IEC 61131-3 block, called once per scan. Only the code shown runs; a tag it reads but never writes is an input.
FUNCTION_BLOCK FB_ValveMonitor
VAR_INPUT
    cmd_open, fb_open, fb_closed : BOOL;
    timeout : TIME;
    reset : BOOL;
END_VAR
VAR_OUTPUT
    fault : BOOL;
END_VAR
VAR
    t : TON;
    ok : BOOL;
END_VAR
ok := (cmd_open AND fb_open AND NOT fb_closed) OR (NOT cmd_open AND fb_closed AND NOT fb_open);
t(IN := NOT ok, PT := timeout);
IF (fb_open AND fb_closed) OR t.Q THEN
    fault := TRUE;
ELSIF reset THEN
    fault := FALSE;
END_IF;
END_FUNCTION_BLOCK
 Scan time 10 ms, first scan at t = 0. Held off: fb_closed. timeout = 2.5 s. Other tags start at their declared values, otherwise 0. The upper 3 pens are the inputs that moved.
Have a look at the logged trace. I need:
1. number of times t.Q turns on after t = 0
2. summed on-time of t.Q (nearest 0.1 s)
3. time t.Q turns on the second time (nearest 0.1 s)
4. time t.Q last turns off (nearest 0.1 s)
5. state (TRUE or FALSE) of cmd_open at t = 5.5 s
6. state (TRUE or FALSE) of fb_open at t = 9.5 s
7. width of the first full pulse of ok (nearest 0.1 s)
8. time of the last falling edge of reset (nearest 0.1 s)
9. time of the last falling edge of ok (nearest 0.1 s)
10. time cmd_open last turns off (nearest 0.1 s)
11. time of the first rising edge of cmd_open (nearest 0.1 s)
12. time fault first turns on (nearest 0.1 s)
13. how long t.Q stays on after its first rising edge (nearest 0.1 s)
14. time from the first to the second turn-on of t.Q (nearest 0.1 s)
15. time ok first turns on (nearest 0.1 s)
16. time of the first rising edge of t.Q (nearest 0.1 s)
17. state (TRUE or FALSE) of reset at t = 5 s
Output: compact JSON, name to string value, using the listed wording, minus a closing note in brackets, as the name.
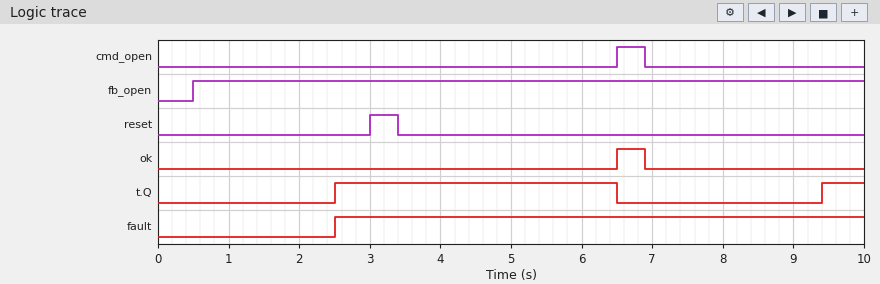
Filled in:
{"number of times t.Q turns on after t = 0": "2", "summed on-time of t.Q": "4.6 s", "time t.Q turns on the second time": "9.4 s", "time t.Q last turns off": "6.5 s", "state (TRUE or FALSE) of cmd_open at t = 5.5 s": "FALSE", "state (TRUE or FALSE) of fb_open at t = 9.5 s": "TRUE", "width of the first full pulse of ok": "0.4 s", "time of the last falling edge of reset": "3.4 s", "time of the last falling edge of ok": "6.9 s", "time cmd_open last turns off": "6.9 s", "time of the first rising edge of cmd_open": "6.5 s", "time fault first turns on": "2.5 s", "how long t.Q stays on after its first rising edge": "4.0 s", "time from the first to the second turn-on of t.Q": "6.9 s", "time ok first turns on": "6.5 s", "time of the first rising edge of t.Q": "2.5 s", "state (TRUE or FALSE) of reset at t = 5 s": "FALSE"}
